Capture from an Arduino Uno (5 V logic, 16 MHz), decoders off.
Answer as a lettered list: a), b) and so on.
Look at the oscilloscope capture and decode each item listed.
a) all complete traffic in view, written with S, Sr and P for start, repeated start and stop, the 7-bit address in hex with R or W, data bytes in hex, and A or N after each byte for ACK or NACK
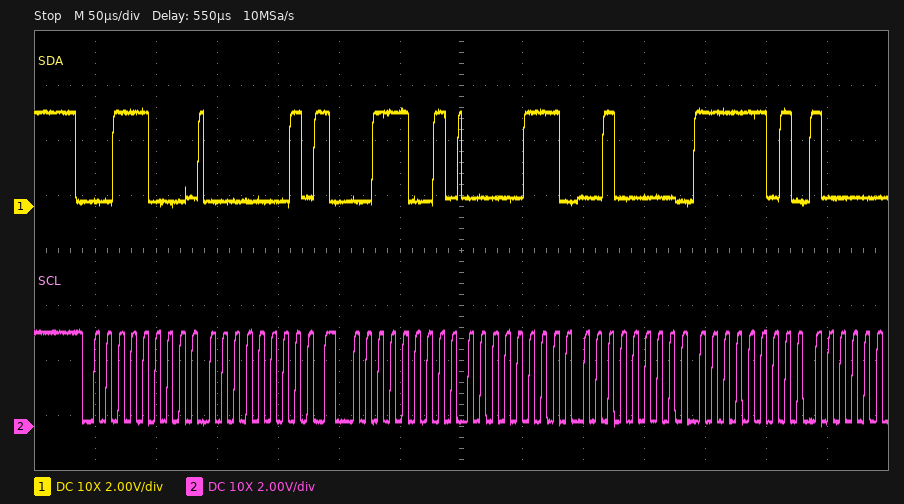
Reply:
a) S 1CW A 01 A Sr 1CR A 07 A 20 A FD A
